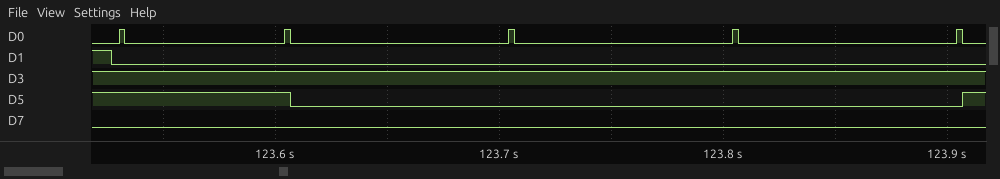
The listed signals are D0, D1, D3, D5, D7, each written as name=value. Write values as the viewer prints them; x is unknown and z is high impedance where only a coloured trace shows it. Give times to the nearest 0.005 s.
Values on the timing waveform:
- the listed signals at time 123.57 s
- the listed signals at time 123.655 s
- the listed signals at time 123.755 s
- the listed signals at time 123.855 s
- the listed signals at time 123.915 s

D0=0, D1=0, D3=1, D5=1, D7=0
D0=0, D1=0, D3=1, D5=0, D7=0
D0=0, D1=0, D3=1, D5=0, D7=0
D0=0, D1=0, D3=1, D5=0, D7=0
D0=0, D1=0, D3=1, D5=1, D7=0
